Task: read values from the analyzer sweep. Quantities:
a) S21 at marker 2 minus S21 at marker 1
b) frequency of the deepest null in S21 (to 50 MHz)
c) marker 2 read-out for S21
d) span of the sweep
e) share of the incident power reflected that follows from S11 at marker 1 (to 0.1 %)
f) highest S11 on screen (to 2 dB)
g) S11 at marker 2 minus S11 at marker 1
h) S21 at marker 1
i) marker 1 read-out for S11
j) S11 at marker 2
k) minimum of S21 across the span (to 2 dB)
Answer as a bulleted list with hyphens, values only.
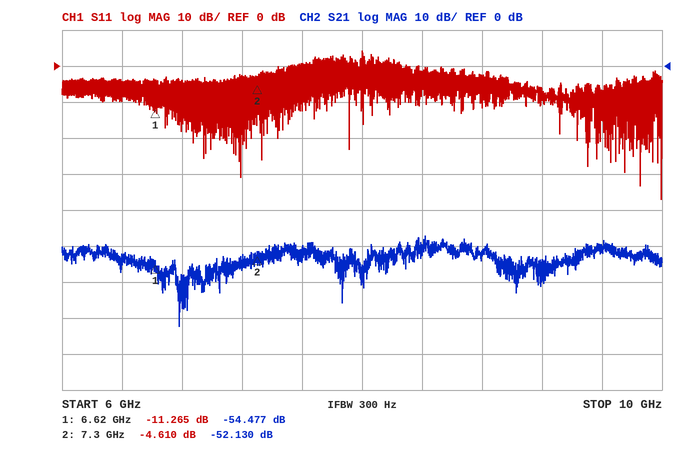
- 2.347 dB
- 6.80 GHz
- -52.130 dB
- 4 GHz
- 7.5 %
- 4 dB
- 6.655 dB
- -54.477 dB
- -11.265 dB
- -4.610 dB
- -72 dB
